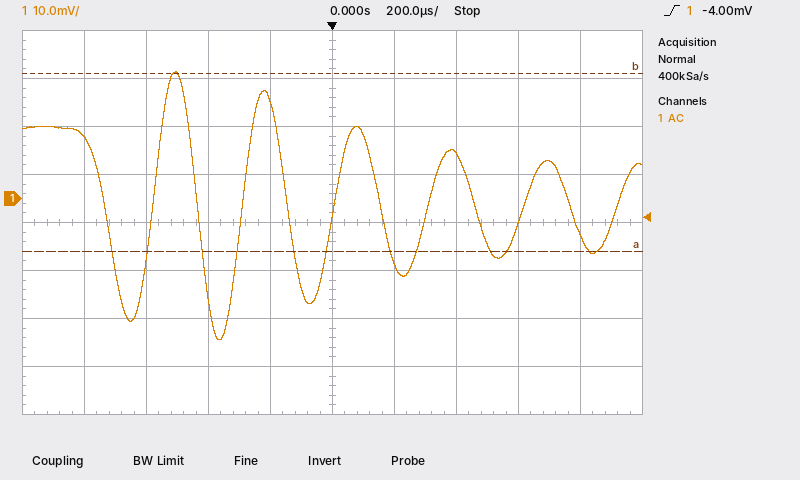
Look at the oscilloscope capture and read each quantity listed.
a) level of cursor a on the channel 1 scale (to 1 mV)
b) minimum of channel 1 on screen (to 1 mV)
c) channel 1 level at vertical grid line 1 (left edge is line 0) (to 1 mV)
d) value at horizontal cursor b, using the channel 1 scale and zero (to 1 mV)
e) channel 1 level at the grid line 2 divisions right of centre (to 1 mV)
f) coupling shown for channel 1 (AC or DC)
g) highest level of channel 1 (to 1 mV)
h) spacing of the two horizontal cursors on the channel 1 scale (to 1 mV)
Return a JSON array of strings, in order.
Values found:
["-11 mV", "-29 mV", "13 mV", "26 mV", "9 mV", "AC", "26 mV", "37 mV"]
